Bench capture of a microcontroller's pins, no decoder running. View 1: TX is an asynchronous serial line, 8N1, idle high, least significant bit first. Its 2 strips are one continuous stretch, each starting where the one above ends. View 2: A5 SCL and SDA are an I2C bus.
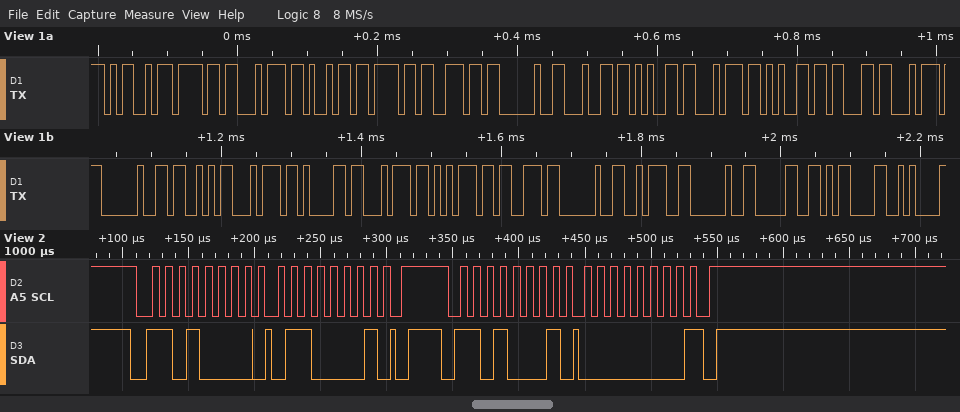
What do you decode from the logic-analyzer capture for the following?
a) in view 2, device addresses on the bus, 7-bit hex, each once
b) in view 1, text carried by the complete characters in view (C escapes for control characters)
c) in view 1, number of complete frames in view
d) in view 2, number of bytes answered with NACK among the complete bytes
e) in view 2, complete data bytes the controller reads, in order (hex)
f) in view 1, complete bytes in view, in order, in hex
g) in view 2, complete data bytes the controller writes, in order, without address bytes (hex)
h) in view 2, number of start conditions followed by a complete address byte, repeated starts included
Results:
0x68
"Motion detect Status : 0\r\n"
26
1
00
4D 6F 74 69 6F 6E 20 64 65 74 65 63 74 20 53 74 61 74 75 73 20 3A 20 30 0D 0A
61
2
